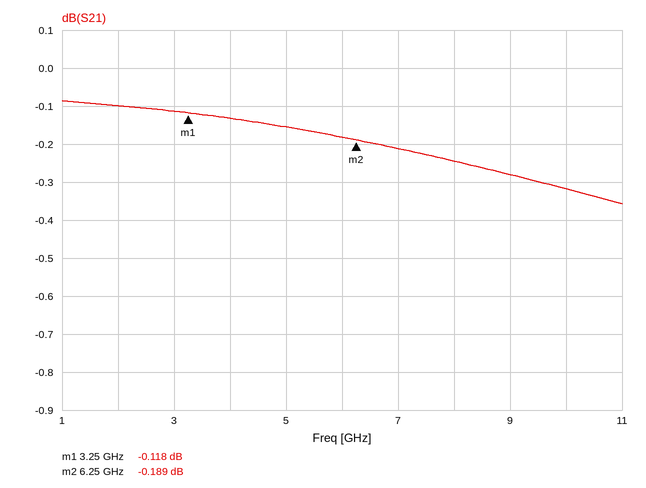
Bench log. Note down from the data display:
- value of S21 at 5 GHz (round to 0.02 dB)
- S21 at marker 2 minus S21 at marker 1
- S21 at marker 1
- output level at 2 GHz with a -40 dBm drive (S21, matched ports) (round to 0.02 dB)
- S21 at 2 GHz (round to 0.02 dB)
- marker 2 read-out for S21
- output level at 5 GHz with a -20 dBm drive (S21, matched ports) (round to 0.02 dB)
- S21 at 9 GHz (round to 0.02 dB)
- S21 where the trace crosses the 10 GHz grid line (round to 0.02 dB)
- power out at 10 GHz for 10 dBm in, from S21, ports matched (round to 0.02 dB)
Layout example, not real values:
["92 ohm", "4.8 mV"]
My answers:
["-0.16 dB", "-0.071 dB", "-0.118 dB", "-40.10 dBm", "-0.10 dB", "-0.189 dB", "-20.16 dBm", "-0.28 dB", "-0.32 dB", "9.68 dBm"]
